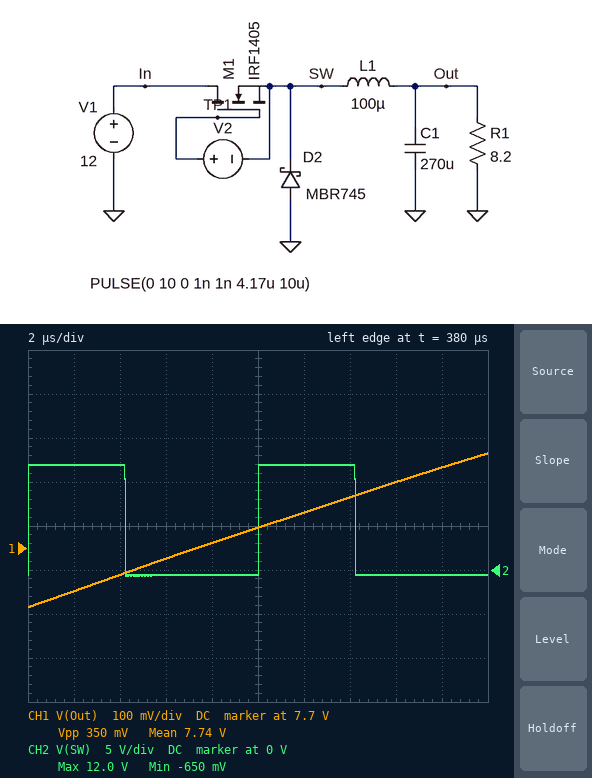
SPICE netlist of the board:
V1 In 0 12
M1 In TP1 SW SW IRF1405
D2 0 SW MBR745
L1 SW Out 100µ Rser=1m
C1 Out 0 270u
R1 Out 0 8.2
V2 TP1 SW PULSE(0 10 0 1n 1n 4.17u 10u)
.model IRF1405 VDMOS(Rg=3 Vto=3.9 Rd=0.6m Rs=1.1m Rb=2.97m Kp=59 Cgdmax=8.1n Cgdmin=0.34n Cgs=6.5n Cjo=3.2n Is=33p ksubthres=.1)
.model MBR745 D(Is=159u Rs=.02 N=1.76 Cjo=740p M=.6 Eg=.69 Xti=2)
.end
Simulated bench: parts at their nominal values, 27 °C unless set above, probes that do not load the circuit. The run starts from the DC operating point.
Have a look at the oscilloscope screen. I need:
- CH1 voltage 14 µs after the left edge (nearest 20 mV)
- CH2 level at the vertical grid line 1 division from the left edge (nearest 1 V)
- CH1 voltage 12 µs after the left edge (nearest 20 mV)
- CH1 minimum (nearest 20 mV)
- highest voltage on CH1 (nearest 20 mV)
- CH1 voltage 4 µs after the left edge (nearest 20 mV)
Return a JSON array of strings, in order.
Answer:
["7.82 V", "12 V", "7.78 V", "7.56 V", "7.92 V", "7.64 V"]
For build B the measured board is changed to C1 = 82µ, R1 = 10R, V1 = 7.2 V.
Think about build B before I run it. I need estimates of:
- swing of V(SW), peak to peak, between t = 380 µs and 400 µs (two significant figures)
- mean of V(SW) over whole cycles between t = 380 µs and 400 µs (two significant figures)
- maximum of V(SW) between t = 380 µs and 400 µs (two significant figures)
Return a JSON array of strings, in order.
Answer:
["8.1 V", "4.6 V", "7.8 V"]
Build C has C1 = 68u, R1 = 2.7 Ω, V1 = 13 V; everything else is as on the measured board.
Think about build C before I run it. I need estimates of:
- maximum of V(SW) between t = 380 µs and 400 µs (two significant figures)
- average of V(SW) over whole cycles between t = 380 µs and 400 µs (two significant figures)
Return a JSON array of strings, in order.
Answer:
["13 V", "5.3 V"]
